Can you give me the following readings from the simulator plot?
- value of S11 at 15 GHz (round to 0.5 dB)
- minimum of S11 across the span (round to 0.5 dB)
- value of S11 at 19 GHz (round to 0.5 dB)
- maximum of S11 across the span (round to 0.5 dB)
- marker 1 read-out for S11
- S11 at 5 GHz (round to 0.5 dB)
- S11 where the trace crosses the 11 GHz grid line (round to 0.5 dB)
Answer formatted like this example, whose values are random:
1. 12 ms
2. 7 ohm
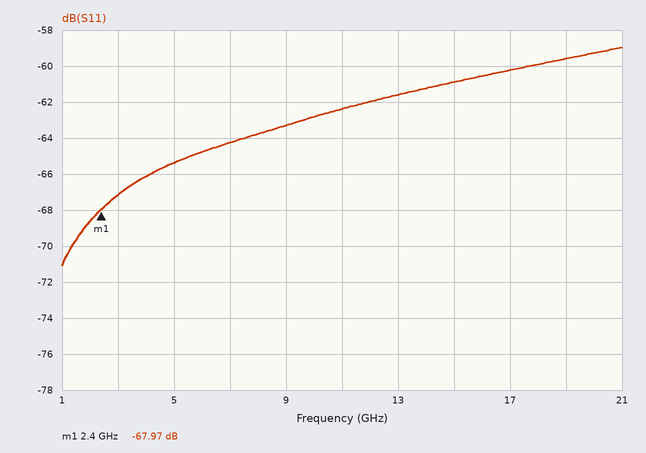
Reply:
1. -61.0 dB
2. -71.0 dB
3. -59.5 dB
4. -59.0 dB
5. -67.97 dB
6. -65.5 dB
7. -62.5 dB
